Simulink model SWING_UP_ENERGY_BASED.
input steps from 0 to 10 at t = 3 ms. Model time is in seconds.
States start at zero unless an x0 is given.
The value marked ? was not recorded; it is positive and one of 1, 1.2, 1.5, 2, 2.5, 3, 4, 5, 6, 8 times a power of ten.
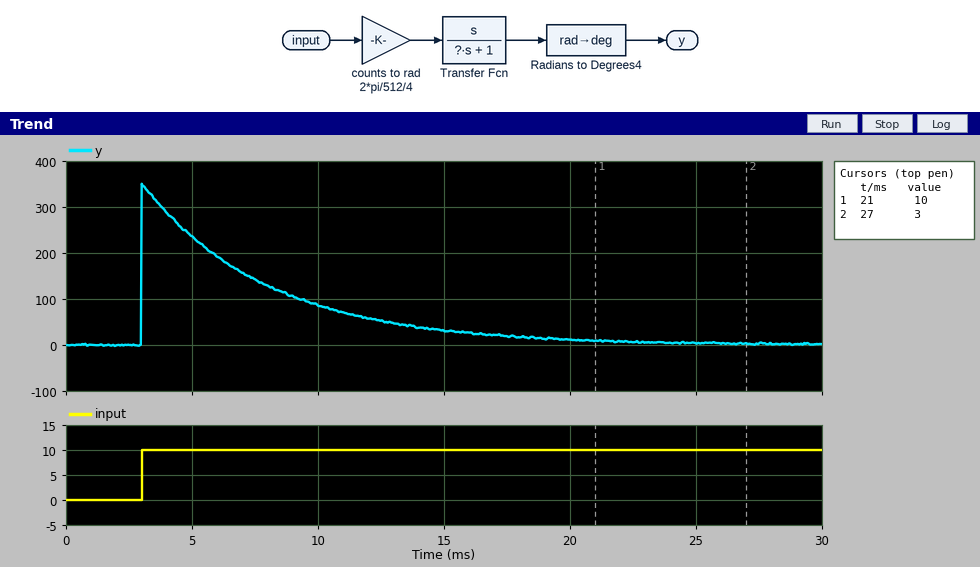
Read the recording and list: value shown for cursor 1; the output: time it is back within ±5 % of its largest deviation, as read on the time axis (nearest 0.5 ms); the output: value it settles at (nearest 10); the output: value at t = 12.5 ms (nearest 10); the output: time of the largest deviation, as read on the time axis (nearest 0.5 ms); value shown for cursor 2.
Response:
10
18.0 ms
0
50
3.0 ms
3
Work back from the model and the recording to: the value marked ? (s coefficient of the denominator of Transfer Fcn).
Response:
0.005
